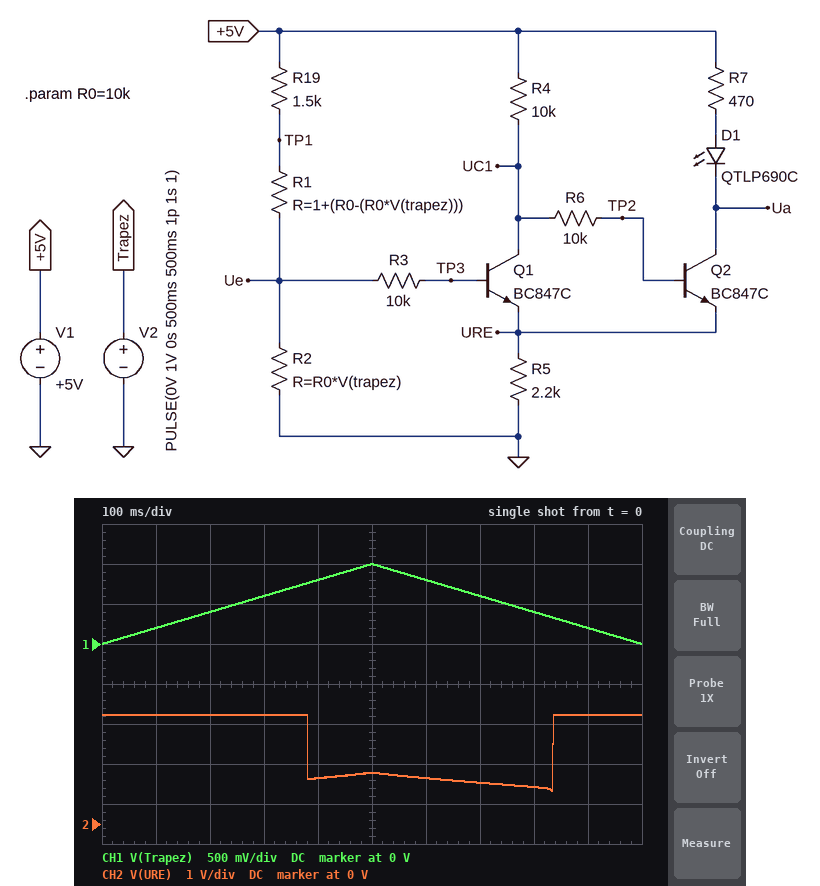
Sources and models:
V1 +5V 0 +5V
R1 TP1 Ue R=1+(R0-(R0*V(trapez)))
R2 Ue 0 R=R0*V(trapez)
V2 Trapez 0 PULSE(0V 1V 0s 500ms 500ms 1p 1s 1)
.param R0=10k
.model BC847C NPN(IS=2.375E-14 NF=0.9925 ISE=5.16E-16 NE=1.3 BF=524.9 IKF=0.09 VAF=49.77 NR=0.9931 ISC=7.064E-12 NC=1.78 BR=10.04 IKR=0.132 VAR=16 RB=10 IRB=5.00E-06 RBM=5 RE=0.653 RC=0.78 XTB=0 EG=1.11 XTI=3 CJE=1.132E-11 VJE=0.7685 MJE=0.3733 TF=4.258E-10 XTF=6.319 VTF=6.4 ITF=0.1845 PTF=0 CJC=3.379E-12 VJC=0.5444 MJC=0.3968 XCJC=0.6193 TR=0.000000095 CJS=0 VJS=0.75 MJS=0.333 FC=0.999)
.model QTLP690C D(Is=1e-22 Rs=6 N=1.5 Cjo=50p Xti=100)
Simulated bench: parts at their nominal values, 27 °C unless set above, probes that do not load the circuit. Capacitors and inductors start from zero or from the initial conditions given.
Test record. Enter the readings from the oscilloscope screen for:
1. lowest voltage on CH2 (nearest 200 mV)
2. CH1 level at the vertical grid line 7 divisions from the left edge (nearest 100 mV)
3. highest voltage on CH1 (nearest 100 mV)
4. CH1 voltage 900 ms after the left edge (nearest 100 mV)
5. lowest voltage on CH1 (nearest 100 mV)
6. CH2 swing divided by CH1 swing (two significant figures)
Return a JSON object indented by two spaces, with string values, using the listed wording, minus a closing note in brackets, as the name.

{
  "lowest voltage on CH2": "800 mV",
  "CH1 level at the vertical grid line 7 divisions from the left edge": "600 mV",
  "highest voltage on CH1": "1.0 V",
  "CH1 voltage 900 ms after the left edge": "200 mV",
  "lowest voltage on CH1": "0 V",
  "CH2 swing divided by CH1 swing": "1.9"
}
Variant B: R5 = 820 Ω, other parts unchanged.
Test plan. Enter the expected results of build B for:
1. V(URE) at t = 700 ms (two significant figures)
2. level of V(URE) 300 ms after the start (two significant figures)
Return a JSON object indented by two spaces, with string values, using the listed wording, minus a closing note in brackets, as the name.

{
  "V(URE) at t = 700 ms": "470 mV",
  "level of V(URE) 300 ms after the start": "2.1 V"
}
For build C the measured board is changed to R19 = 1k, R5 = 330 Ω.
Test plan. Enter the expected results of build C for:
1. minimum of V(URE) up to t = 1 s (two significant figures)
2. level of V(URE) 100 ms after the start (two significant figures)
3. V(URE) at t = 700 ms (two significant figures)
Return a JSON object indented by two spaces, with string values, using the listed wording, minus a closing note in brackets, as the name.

{
  "minimum of V(URE) up to t = 1 s": "150 mV",
  "level of V(URE) 100 ms after the start": "1.3 V",
  "V(URE) at t = 700 ms": "210 mV"
}
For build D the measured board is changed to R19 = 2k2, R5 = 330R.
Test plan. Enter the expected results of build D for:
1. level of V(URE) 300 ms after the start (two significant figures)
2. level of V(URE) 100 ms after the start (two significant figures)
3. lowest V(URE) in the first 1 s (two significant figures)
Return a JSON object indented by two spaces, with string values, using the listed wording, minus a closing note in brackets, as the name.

{
  "level of V(URE) 300 ms after the start": "200 mV",
  "level of V(URE) 100 ms after the start": "1.3 V",
  "lowest V(URE) in the first 1 s": "150 mV"
}
